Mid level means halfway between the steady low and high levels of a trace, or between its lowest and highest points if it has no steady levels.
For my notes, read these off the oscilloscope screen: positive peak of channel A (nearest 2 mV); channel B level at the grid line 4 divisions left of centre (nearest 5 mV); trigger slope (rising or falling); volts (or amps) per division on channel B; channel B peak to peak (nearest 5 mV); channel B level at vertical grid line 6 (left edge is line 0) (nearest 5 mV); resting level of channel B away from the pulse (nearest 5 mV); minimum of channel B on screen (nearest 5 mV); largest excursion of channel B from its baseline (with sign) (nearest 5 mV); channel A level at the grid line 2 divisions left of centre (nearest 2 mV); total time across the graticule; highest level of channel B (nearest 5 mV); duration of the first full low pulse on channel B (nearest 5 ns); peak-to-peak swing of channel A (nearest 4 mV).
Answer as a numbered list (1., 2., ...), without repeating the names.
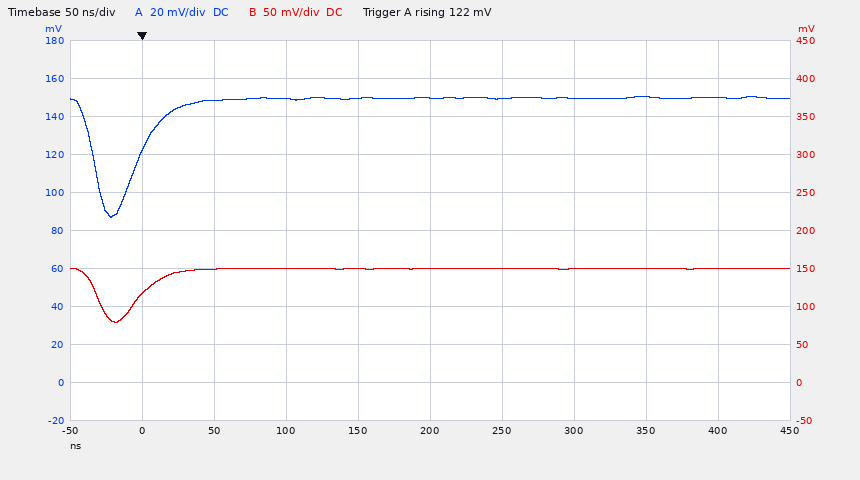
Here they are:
1. 150 mV
2. 115 mV
3. rising
4. 50 mV
5. 70 mV
6. 150 mV
7. 150 mV
8. 80 mV
9. -70 mV
10. 150 mV
11. 500 ns
12. 150 mV
13. 30 ns
14. 64 mV
